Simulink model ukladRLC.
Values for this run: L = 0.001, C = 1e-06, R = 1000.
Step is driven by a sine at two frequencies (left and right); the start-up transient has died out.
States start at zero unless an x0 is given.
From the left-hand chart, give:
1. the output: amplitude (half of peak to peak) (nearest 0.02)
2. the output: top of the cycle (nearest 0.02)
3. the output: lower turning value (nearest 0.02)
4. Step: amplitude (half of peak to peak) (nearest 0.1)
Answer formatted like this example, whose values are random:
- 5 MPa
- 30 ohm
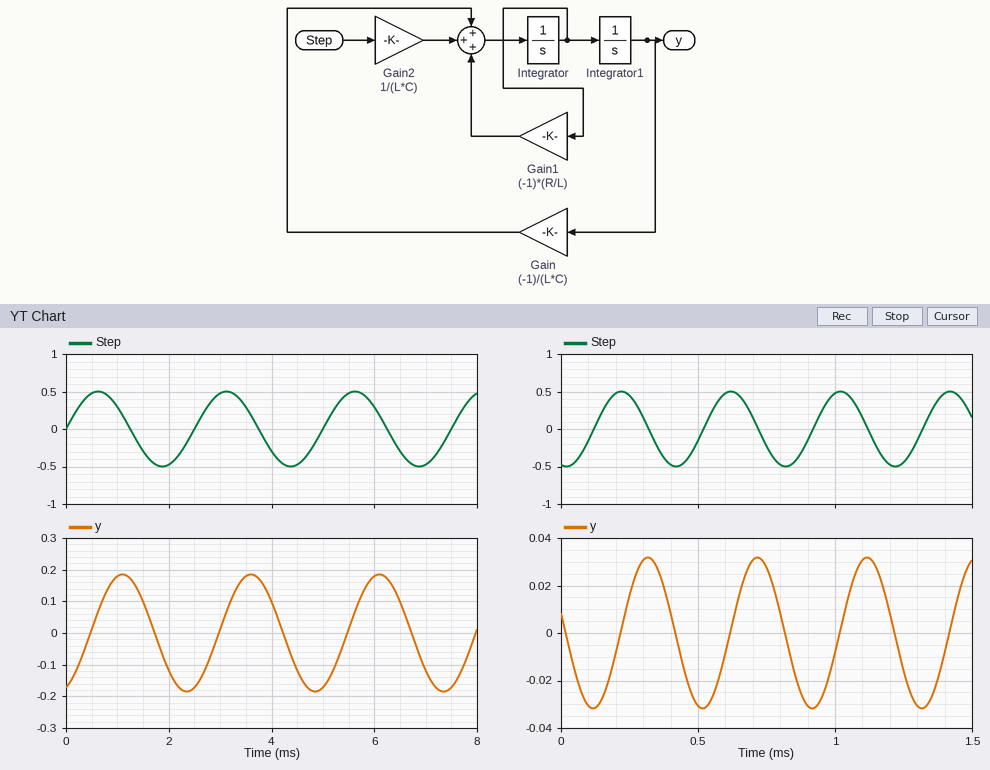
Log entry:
- 0.18
- 0.18
- -0.18
- 0.5
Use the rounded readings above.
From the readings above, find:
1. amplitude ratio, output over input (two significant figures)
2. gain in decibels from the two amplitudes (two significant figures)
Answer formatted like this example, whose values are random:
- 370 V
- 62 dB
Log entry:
- 0.36
- -8.9 dB
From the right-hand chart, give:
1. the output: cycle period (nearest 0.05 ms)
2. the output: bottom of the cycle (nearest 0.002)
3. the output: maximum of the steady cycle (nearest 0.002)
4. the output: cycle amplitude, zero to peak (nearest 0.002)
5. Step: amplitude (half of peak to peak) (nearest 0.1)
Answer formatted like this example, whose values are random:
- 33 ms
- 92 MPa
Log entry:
- 0.40 ms
- -0.032
- 0.032
- 0.032
- 0.5
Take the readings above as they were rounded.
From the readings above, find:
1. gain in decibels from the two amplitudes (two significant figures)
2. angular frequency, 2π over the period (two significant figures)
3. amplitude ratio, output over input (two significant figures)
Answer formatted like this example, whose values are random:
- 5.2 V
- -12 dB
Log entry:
- -24 dB
- 16 rad/ms
- 0.064
